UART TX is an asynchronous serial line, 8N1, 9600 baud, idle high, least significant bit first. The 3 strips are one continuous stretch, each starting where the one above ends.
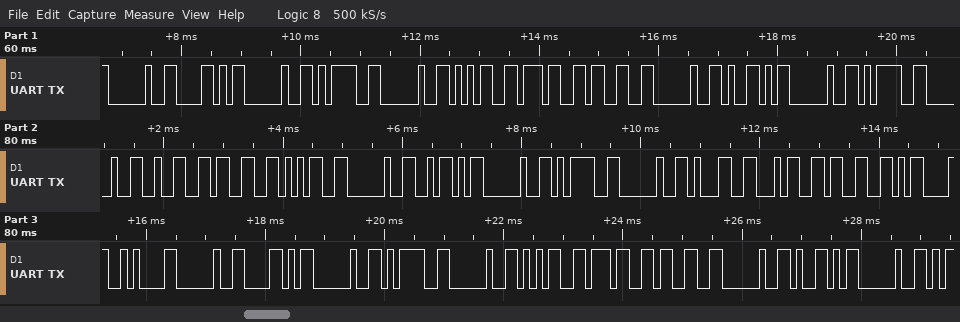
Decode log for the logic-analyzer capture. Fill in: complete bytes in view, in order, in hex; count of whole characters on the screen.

20 58 20 3D 20 35 37 33 20 59 20 3D 20 32 33 35 20 5A 20 3D 20 31 34 33 0D 0A 20 58 20 3D 20 35 37 33 20 59 20
37
